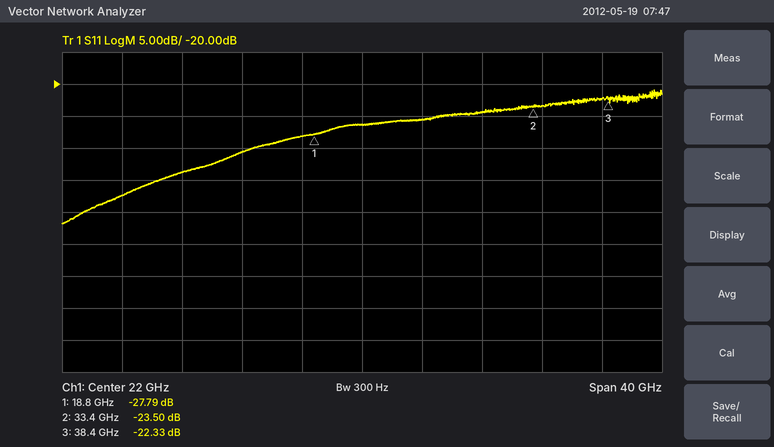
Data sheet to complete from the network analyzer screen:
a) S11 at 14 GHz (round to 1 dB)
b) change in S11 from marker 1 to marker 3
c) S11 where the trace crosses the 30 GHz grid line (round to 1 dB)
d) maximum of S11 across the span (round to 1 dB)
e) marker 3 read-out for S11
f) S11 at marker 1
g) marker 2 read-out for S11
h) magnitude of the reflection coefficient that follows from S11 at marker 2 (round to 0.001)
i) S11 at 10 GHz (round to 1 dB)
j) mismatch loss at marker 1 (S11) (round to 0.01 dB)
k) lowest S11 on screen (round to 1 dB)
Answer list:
-31 dB
5.46 dB
-24 dB
-21 dB
-22.33 dB
-27.79 dB
-23.50 dB
0.067
-34 dB
0.01 dB
-42 dB
